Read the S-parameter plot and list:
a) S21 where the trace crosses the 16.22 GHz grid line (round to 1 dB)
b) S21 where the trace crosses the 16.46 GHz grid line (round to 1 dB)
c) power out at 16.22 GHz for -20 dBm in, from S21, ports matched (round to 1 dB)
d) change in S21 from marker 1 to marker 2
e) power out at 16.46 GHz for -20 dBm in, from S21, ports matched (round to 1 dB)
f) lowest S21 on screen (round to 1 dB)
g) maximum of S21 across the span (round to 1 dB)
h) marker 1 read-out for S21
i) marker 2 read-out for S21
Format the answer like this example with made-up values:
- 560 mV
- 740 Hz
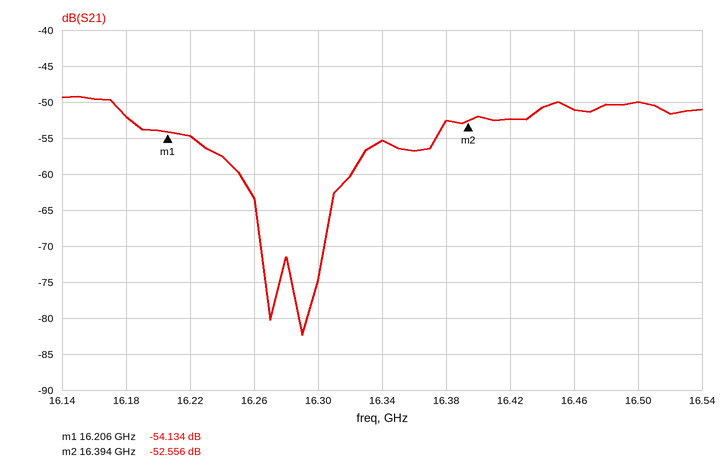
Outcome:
- -55 dB
- -51 dB
- -75 dBm
- 1.578 dB
- -71 dBm
- -82 dB
- -49 dB
- -54.134 dB
- -52.556 dB
